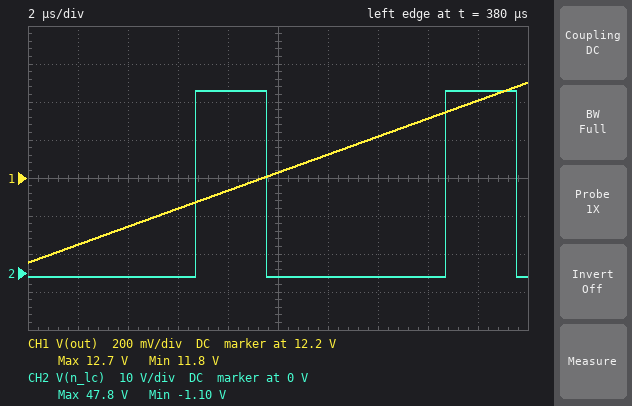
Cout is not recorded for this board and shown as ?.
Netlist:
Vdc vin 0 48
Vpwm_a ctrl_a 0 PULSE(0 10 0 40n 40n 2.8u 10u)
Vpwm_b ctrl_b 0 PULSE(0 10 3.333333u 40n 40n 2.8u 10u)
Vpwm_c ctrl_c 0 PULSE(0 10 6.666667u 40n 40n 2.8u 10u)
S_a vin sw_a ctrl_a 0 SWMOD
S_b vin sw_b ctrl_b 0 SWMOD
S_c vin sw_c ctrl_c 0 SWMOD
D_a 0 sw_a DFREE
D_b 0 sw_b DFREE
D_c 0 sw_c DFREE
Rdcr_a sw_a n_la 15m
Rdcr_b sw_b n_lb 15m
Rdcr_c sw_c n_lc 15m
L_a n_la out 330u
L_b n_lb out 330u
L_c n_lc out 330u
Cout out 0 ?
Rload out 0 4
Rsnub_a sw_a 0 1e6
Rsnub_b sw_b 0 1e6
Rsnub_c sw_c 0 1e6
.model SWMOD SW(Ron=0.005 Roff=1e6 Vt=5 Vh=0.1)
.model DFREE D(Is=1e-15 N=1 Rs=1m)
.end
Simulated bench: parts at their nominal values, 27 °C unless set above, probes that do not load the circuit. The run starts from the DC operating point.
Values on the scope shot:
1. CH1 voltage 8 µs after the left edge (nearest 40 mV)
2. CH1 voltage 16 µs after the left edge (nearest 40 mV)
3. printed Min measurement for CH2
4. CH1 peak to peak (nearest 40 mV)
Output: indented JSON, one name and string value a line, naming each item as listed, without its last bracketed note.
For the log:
{
  "CH1 voltage 8 µs after the left edge": "12.12 V",
  "CH1 voltage 16 µs after the left edge": "12.52 V",
  "printed Min measurement for CH2": "-1.10 V",
  "CH1 peak to peak": "960 mV"
}
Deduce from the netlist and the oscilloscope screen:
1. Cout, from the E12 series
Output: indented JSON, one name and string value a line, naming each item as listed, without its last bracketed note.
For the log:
{
  "Cout, from the E12 series": "560 µF"
}
